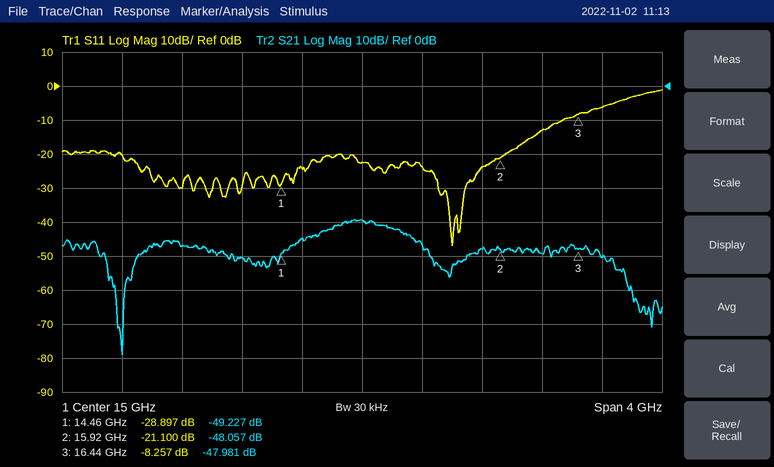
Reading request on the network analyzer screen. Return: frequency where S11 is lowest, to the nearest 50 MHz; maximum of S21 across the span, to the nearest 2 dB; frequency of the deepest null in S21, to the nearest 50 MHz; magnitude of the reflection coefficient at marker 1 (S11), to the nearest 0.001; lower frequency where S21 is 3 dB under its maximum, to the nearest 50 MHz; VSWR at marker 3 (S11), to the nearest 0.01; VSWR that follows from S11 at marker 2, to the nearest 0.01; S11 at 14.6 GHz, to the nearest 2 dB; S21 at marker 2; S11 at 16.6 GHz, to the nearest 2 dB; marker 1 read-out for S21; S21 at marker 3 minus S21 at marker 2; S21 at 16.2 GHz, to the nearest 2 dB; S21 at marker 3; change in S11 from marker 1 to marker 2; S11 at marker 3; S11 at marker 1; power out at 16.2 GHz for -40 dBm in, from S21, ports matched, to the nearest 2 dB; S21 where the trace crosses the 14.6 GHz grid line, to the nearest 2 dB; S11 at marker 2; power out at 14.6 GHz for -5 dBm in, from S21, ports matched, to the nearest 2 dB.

15.60 GHz
-40 dB
13.40 GHz
0.036
14.75 GHz
2.26
1.19
-24 dB
-48.057 dB
-6 dB
-49.227 dB
0.076 dB
-50 dB
-47.981 dB
7.797 dB
-8.257 dB
-28.897 dB
-90 dBm
-44 dB
-21.100 dB
-50 dBm
